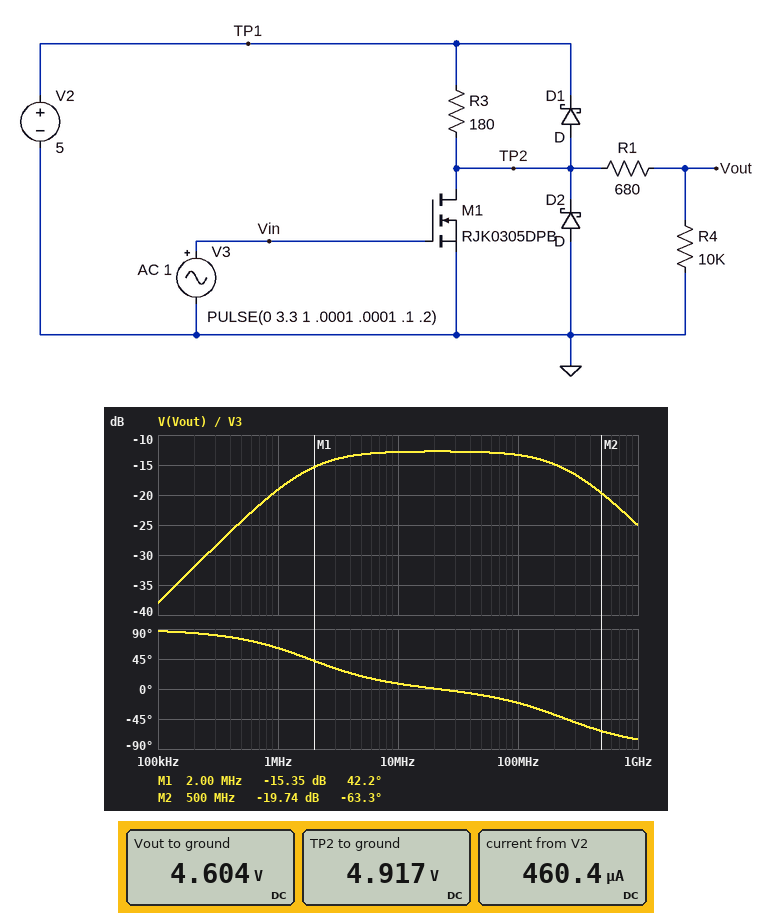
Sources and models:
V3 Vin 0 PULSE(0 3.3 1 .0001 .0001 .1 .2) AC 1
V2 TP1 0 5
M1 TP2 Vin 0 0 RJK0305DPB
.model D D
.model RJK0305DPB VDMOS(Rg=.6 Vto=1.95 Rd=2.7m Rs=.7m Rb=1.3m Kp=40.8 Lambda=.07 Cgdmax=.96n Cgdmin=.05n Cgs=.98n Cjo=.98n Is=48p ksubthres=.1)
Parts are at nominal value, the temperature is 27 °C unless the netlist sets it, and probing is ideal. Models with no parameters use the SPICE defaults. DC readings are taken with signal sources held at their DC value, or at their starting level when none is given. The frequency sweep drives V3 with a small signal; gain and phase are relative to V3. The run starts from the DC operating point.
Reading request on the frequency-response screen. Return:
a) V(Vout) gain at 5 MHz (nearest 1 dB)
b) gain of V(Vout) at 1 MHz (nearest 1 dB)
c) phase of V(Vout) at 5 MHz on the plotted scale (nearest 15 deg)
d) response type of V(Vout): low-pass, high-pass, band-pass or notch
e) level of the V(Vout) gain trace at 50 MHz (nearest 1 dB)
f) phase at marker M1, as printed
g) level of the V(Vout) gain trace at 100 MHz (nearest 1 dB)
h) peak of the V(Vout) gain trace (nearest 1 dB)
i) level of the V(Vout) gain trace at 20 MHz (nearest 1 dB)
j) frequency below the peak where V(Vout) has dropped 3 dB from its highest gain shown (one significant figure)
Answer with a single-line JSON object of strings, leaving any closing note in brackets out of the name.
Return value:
{"V(Vout) gain at 5 MHz": "-13 dB", "gain of V(Vout) at 1 MHz": "-19 dB", "phase of V(Vout) at 5 MHz on the plotted scale": "15 deg", "response type of V(Vout): low-pass, high-pass, band-pass or notch": "band-pass", "level of the V(Vout) gain trace at 50 MHz": "-13 dB", "phase at marker M1, as printed": "42.2 deg", "level of the V(Vout) gain trace at 100 MHz": "-13 dB", "peak of the V(Vout) gain trace": "-13 dB", "level of the V(Vout) gain trace at 20 MHz": "-13 dB", "frequency below the peak where V(Vout) has dropped 3 dB from its highest gain shown": "2 MHz"}
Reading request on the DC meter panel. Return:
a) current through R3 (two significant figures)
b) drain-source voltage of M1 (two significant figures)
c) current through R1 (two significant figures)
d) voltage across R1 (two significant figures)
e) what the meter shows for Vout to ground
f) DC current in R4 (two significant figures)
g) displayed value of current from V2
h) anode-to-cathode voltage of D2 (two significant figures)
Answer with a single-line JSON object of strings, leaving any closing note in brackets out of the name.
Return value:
{"current through R3": "460 µA", "drain-source voltage of M1": "4.9 V", "current through R1": "460 µA", "voltage across R1": "310 mV", "what the meter shows for Vout to ground": "4.604 V", "DC current in R4": "460 µA", "displayed value of current from V2": "460.4 µA", "anode-to-cathode voltage of D2": "-4.9 V"}
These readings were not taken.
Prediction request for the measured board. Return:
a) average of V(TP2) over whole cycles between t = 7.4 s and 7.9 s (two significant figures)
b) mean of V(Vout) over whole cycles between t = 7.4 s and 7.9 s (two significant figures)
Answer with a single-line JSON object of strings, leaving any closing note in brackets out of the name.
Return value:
{"average of V(TP2) over whole cycles between t = 7.4 s and 7.9 s": "2.5 V", "mean of V(Vout) over whole cycles between t = 7.4 s and 7.9 s": "2.3 V"}
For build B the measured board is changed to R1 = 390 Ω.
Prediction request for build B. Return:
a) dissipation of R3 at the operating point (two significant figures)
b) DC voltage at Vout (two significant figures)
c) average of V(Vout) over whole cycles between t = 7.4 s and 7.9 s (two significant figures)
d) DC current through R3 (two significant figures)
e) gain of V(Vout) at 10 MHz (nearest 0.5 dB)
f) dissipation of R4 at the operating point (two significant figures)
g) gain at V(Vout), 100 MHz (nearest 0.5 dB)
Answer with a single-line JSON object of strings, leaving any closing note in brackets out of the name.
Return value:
{"dissipation of R3 at the operating point": "40 µW", "DC voltage at Vout": "4.7 V", "average of V(Vout) over whole cycles between t = 7.4 s and 7.9 s": "2.4 V", "DC current through R3": "470 µA", "gain of V(Vout) at 10 MHz": "-12.5 dB", "dissipation of R4 at the operating point": "2.2 mW", "gain at V(Vout), 100 MHz": "-13.0 dB"}
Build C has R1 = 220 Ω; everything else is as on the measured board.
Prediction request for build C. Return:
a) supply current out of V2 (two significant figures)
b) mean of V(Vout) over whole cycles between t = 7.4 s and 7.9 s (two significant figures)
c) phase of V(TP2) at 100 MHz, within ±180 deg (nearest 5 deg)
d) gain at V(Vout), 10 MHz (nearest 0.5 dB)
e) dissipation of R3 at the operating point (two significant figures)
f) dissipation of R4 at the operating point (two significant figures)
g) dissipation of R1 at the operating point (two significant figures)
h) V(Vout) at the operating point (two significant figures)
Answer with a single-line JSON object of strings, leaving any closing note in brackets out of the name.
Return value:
{"supply current out of V2": "480 µA", "mean of V(Vout) over whole cycles between t = 7.4 s and 7.9 s": "2.4 V", "phase of V(TP2) at 100 MHz, within ±180 deg": "-20 deg", "gain at V(Vout), 10 MHz": "-12.5 dB", "dissipation of R3 at the operating point": "42 µW", "dissipation of R4 at the operating point": "2.3 mW", "dissipation of R1 at the operating point": "51 µW", "V(Vout) at the operating point": "4.8 V"}
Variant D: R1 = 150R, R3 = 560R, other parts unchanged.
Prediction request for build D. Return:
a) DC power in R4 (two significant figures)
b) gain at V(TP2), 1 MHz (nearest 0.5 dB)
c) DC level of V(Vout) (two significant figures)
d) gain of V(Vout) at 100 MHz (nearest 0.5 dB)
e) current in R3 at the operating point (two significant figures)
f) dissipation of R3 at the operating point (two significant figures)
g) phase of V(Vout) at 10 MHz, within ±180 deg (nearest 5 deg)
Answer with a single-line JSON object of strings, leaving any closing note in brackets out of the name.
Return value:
{"DC power in R4": "2.2 mW", "gain at V(TP2), 1 MHz": "-13.5 dB", "DC level of V(Vout)": "4.7 V", "gain of V(Vout) at 100 MHz": "-13.0 dB", "current in R3 at the operating point": "470 µA", "dissipation of R3 at the operating point": "120 µW", "phase of V(Vout) at 10 MHz, within ±180 deg": "0 deg"}
